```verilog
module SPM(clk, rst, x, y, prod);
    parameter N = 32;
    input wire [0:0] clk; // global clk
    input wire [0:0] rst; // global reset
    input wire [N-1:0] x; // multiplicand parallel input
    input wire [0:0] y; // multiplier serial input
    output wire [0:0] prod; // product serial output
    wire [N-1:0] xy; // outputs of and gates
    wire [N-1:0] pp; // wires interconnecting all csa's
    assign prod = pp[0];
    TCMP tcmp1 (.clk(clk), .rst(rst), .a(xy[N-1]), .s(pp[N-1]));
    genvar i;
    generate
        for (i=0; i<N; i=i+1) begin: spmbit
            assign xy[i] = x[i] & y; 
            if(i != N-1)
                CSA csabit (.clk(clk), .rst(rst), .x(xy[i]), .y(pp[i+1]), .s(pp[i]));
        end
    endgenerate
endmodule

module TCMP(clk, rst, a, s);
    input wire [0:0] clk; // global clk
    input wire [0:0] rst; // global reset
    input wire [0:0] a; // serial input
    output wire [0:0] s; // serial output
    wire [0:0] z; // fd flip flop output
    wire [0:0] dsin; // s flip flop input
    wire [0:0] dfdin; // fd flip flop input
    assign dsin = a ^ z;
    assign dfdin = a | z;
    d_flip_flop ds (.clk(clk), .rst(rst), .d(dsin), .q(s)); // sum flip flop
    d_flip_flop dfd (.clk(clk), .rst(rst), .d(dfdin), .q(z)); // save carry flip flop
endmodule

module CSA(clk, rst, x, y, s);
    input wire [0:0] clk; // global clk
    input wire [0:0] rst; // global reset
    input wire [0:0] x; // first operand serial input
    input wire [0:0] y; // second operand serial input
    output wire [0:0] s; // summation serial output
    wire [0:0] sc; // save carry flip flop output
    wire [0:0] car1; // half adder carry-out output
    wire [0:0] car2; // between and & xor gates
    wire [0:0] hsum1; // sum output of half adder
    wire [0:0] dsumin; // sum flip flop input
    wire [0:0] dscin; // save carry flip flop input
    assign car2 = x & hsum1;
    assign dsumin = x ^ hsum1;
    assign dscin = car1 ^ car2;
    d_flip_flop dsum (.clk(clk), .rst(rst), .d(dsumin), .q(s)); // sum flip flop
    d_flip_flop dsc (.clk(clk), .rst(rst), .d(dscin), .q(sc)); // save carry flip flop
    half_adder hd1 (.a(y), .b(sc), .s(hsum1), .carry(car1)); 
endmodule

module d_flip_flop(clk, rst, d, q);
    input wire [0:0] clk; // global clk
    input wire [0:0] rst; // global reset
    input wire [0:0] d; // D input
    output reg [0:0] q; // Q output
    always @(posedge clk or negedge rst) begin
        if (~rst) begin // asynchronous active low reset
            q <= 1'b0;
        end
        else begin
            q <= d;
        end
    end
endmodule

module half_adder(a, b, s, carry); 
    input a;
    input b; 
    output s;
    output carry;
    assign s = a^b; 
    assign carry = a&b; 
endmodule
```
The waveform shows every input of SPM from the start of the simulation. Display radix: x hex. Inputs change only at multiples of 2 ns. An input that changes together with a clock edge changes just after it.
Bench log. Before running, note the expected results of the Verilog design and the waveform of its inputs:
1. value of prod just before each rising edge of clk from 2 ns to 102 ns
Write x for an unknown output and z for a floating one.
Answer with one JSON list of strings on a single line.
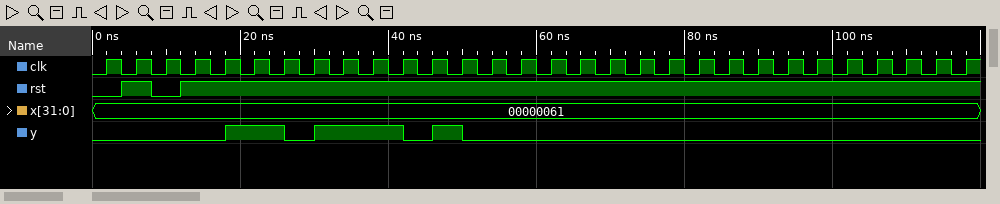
["0 0 0 0 0 0 1 1 0 1 1 0 1 1 0 1 1 0 0 0 1 0 0 0 0 0"]
